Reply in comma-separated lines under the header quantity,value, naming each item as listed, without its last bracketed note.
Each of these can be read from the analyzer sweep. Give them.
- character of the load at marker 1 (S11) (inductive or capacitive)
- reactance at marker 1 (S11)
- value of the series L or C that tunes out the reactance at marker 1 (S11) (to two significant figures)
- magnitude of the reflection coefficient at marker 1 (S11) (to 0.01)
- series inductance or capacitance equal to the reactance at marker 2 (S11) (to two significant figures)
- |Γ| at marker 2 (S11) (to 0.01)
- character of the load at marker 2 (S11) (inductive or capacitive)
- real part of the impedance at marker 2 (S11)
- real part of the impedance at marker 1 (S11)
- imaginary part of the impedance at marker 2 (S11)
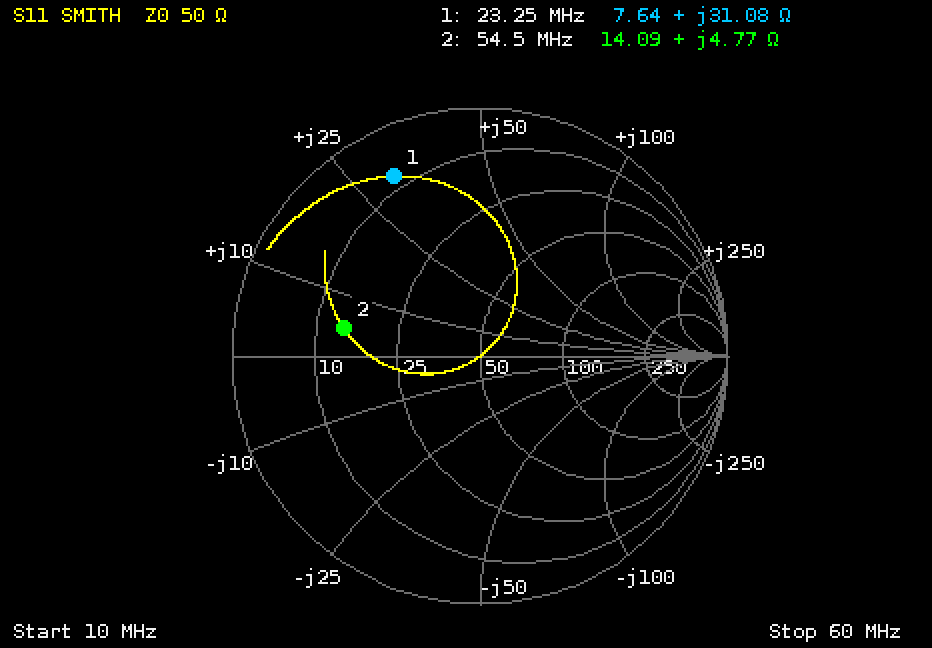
quantity,value
character of the load at marker 1 (S11),inductive
reactance at marker 1,+31.08 Ω
value of the series L or C that tunes out the reactance at marker 1 (S11),220 pF
magnitude of the reflection coefficient at marker 1 (S11),0.80
series inductance or capacitance equal to the reactance at marker 2 (S11),14 nH
|Γ| at marker 2 (S11),0.56
character of the load at marker 2 (S11),inductive
real part of the impedance at marker 2,14.09 Ω
real part of the impedance at marker 1,7.64 Ω
imaginary part of the impedance at marker 2,+4.77 Ω
